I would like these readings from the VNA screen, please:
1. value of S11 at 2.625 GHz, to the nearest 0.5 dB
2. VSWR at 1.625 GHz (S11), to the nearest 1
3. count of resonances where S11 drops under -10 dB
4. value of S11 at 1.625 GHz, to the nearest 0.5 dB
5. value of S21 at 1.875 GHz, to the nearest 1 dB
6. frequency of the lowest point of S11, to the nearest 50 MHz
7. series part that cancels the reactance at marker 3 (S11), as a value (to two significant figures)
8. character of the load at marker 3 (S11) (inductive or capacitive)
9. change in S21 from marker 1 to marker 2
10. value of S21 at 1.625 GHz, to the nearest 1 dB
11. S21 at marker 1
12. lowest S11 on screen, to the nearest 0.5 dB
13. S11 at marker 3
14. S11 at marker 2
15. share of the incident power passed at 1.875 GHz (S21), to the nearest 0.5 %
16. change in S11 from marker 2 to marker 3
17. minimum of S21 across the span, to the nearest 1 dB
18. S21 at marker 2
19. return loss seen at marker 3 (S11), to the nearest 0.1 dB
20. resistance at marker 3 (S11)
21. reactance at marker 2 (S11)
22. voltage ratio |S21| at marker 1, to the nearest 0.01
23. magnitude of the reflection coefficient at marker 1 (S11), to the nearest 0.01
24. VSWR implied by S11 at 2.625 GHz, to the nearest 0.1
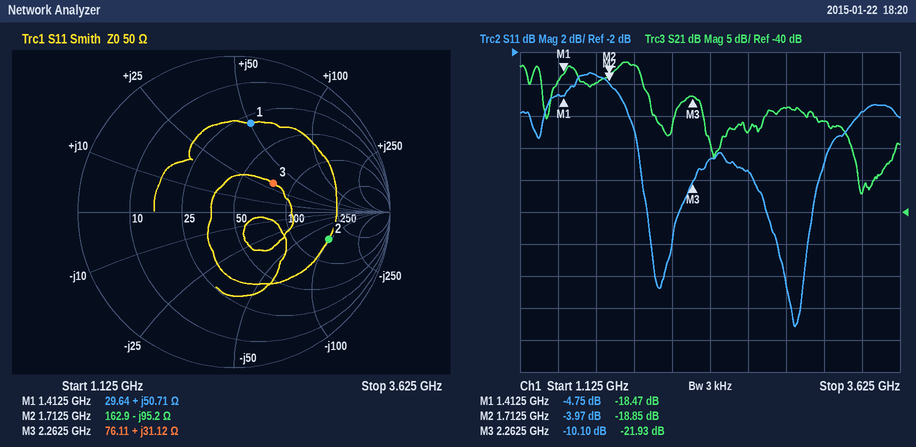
-9.5 dB
5
2
-3.5 dB
-17 dB
2.95 GHz
2.3 pF
inductive
-0.38 dB
-20 dB
-18.47 dB
-19.0 dB
-10.10 dB
-3.97 dB
2.0 %
-6.13 dB
-37 dB
-18.85 dB
10.1 dB
76.11 Ω
-95.2 Ω
0.12
0.58
2.0
